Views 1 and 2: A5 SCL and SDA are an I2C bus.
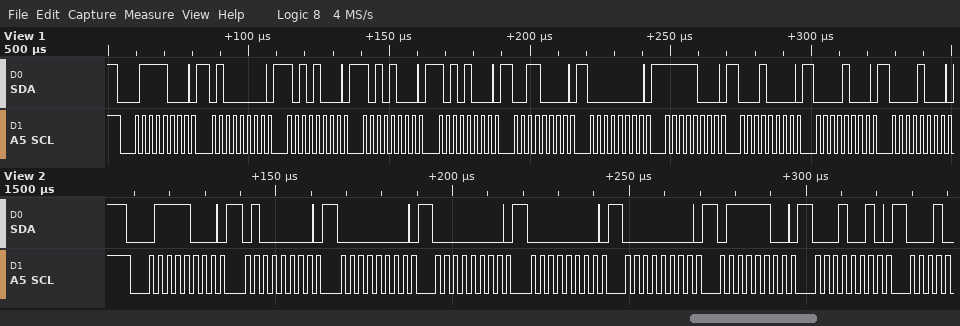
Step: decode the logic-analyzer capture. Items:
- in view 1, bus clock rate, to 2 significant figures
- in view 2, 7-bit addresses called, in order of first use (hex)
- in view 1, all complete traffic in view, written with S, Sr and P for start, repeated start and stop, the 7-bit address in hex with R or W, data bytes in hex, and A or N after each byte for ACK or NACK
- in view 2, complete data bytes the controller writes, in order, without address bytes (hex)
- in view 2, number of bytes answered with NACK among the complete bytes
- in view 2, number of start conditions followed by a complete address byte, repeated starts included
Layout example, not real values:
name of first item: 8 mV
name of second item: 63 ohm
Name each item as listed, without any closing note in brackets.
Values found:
in view 1, bus clock rate, to 2 significant figures: 400 kHz
in view 2, 7-bit addresses called, in order of first use: 0x3C
in view 1, all complete traffic in view, written with S, Sr and P for start, repeated start and stop, the 7-bit address in hex with R or W, data bytes in hex, and A or N after each byte for ACK or NACK: S 3CW A 40 A A8 A A8 A A8 A 30 A 00 A F8 A 10 A 08 A 08 A
in view 2, complete data bytes the controller writes, in order, without address bytes: 40 00 00 00 00 7C 12
in view 2, number of bytes answered with NACK among the complete bytes: 0
in view 2, number of start conditions followed by a complete address byte, repeated starts included: 1
